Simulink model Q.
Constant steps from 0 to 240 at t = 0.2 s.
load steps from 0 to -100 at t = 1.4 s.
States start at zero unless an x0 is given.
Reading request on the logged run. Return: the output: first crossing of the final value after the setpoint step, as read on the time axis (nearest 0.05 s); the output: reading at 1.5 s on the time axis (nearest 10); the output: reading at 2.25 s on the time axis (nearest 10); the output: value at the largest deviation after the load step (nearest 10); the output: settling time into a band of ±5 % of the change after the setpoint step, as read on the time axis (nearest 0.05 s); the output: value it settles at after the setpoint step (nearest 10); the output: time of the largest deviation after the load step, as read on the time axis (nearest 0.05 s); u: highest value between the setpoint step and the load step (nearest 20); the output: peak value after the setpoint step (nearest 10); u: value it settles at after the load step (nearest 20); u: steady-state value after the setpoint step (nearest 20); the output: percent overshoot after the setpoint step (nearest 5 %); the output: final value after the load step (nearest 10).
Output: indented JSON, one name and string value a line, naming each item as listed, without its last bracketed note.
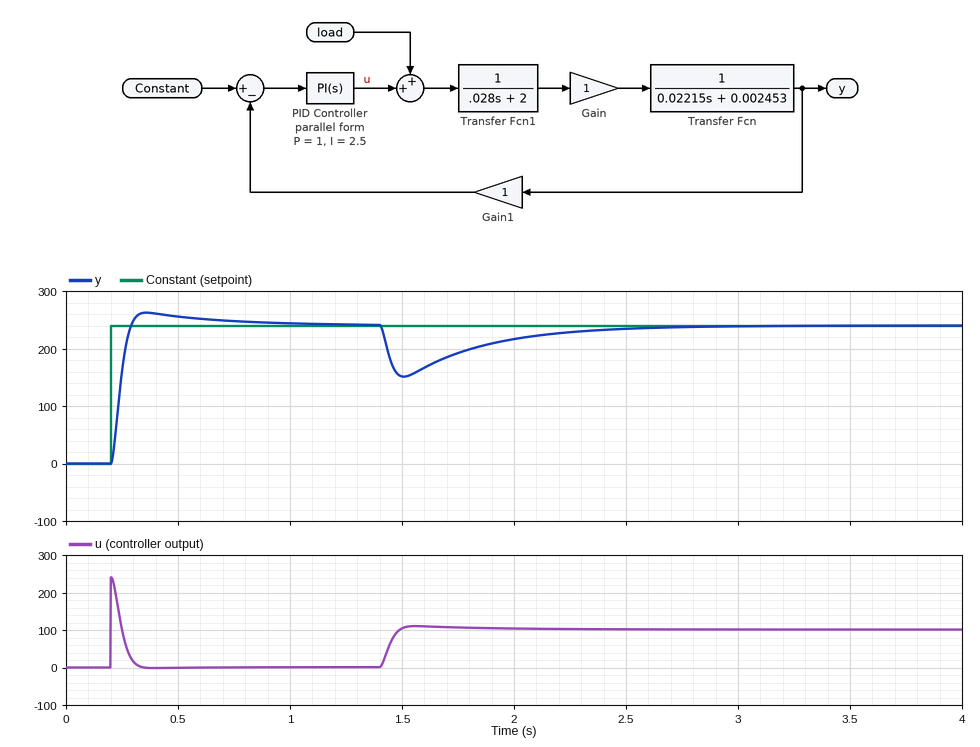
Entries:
{
  "the output: first crossing of the final value after the setpoint step, as read on the time axis": "0.30 s",
  "the output: reading at 1.5 s on the time axis": "150",
  "the output: reading at 2.25 s on the time axis": "230",
  "the output: value at the largest deviation after the load step": "150",
  "the output: settling time into a band of ±5 % of the change after the setpoint step, as read on the time axis": "0.60 s",
  "the output: value it settles at after the setpoint step": "240",
  "the output: time of the largest deviation after the load step, as read on the time axis": "1.50 s",
  "u: highest value between the setpoint step and the load step": "240",
  "the output: peak value after the setpoint step": "260",
  "u: value it settles at after the load step": "100",
  "u: steady-state value after the setpoint step": "0",
  "the output: percent overshoot after the setpoint step": "10 %",
  "the output: final value after the load step": "240"
}
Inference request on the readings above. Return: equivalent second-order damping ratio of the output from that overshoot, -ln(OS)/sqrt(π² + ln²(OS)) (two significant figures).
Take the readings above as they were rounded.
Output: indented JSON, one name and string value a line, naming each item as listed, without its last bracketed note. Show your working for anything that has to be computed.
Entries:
{
  "equivalent second-order damping ratio of the output from that overshoot, -ln(OS)/sqrt(π² + ln²(OS))": "ln(0.1) = -2.303; 2.303 / sqrt(9.870 + 5.302) = 0.59"
}
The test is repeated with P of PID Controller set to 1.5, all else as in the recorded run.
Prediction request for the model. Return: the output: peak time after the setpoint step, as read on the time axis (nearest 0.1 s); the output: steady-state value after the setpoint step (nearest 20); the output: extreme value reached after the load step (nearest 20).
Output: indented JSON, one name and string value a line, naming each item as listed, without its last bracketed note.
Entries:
{
  "the output: peak time after the setpoint step, as read on the time axis": "0.3 s",
  "the output: steady-state value after the setpoint step": "240",
  "the output: extreme value reached after the load step": "180"
}
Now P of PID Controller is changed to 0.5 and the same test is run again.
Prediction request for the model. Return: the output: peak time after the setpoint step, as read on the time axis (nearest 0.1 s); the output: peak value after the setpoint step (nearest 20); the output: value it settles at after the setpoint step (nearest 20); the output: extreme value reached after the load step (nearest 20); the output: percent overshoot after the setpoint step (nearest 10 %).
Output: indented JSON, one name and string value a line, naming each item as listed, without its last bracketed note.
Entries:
{
  "the output: peak time after the setpoint step, as read on the time axis": "0.5 s",
  "the output: peak value after the setpoint step": "300",
  "the output: value it settles at after the setpoint step": "240",
  "the output: extreme value reached after the load step": "100",
  "the output: percent overshoot after the setpoint step": "20 %"
}
